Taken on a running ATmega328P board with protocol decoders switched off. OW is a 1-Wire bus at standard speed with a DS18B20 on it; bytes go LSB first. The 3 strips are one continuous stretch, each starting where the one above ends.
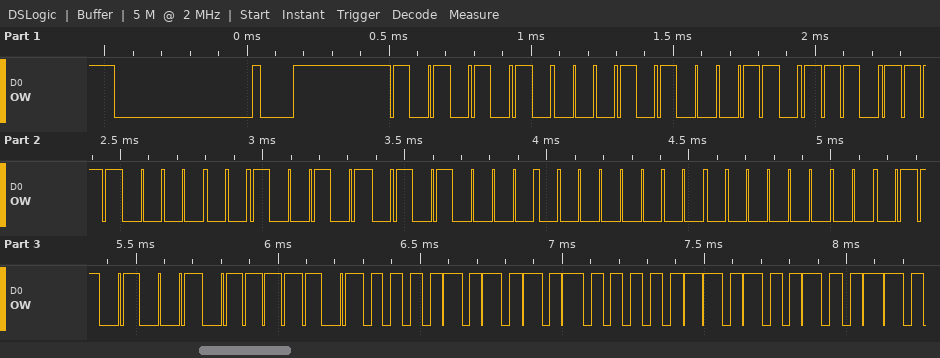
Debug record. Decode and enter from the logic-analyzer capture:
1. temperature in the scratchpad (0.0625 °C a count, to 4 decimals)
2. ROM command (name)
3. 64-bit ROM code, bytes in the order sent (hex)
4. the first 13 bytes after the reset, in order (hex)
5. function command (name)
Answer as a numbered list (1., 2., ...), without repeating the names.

1. 85.0000 °C
2. Match ROM
3. 28 76 0F A4 0A 00 00 96
4. 55 28 76 0F A4 0A 00 00 96 BE 50 05 4B
5. Read Scratchpad
